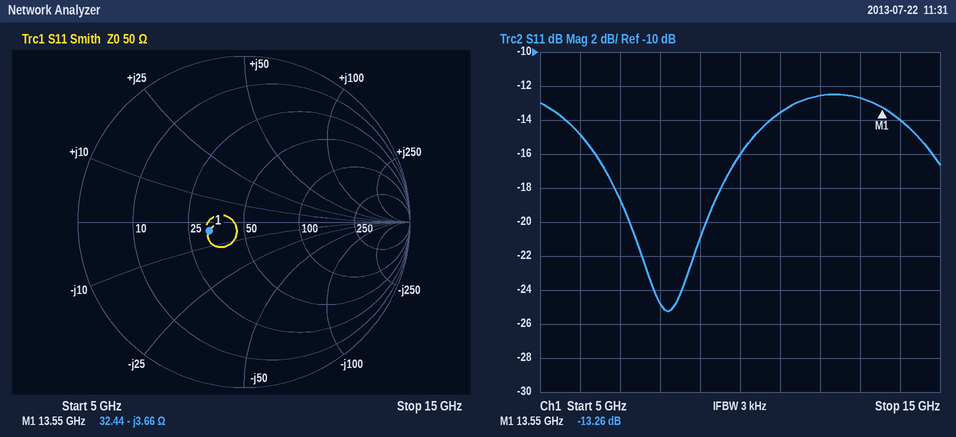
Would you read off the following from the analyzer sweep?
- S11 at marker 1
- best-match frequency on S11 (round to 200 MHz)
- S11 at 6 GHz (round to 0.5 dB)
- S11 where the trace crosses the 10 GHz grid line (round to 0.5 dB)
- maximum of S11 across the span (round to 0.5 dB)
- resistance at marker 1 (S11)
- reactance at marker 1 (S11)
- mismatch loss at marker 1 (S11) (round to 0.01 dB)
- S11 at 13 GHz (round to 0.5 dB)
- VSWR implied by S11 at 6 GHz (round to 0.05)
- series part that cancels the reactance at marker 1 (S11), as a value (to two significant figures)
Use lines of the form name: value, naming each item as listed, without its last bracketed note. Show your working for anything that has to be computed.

S11 at marker 1: -13.26 dB
best-match frequency on S11: 8.2 GHz
S11 at 6 GHz: -15.0 dB
S11 where the trace crosses the 10 GHz grid line: -16.0 dB
maximum of S11 across the span: -12.5 dB
resistance at marker 1: 32.44 Ω
reactance at marker 1: -3.66 Ω
mismatch loss at marker 1 (S11): −10 log10(1 − 10^(-13.26/10)) ≈ 0.21 dB
S11 at 13 GHz: -12.5 dB
VSWR implied by S11 at 6 GHz: |Γ| = 10^(-15/20) = 0.1778; VSWR = (1 + 0.1778)/(1 − 0.1778) ≈ 1.43, so 1.45 to the nearest 0.05
series part that cancels the reactance at marker 1 (S11), as a value: L = 3.66 Ω/(2π × 13.55 GHz) ≈ 43 pH
